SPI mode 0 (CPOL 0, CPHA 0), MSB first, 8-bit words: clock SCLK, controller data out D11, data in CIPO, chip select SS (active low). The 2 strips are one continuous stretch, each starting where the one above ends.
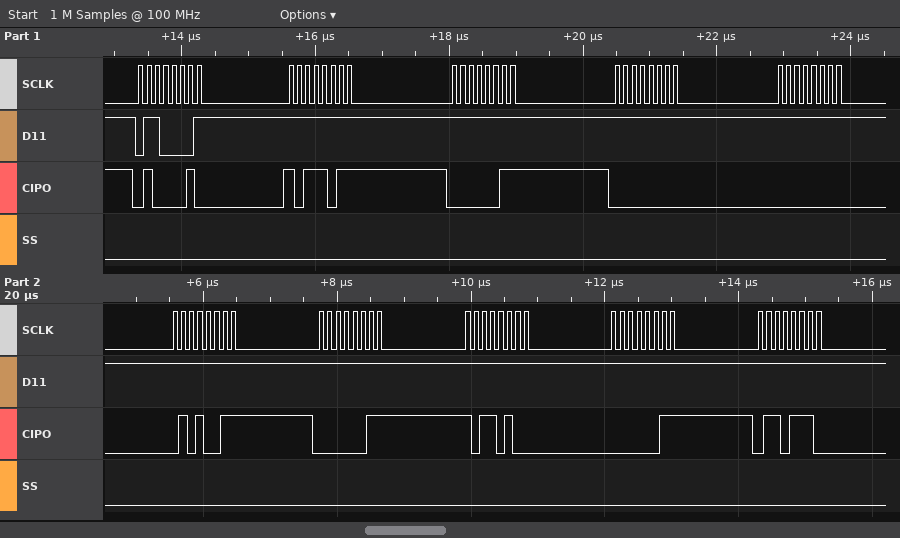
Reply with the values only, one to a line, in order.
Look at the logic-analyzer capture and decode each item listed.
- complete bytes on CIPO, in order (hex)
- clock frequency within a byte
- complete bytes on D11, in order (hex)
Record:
0x42 0xBB 0x03 0x00 0x00 0x53 0x03 0xB4 0x03 0x6E
8 MHz
0x61 0xFF 0xFF 0xFF 0xFF 0xFF 0xFF 0xFF 0xFF 0xFF
